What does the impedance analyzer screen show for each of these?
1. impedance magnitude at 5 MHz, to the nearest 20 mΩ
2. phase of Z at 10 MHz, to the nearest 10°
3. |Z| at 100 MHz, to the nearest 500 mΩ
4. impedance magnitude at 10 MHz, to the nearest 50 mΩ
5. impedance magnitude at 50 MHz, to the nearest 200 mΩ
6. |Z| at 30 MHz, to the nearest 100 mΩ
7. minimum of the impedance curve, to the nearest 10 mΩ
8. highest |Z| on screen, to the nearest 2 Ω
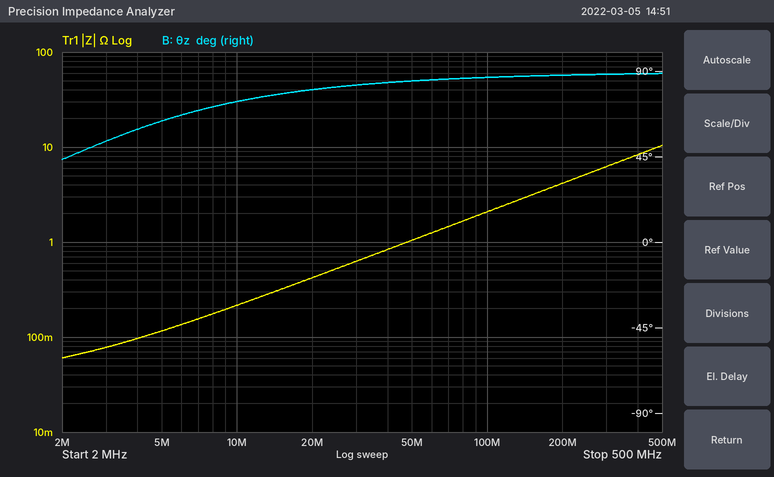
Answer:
120 mΩ
70°
2.0 Ω
200 mΩ
1.0 Ω
600 mΩ
60 mΩ
10 Ω
